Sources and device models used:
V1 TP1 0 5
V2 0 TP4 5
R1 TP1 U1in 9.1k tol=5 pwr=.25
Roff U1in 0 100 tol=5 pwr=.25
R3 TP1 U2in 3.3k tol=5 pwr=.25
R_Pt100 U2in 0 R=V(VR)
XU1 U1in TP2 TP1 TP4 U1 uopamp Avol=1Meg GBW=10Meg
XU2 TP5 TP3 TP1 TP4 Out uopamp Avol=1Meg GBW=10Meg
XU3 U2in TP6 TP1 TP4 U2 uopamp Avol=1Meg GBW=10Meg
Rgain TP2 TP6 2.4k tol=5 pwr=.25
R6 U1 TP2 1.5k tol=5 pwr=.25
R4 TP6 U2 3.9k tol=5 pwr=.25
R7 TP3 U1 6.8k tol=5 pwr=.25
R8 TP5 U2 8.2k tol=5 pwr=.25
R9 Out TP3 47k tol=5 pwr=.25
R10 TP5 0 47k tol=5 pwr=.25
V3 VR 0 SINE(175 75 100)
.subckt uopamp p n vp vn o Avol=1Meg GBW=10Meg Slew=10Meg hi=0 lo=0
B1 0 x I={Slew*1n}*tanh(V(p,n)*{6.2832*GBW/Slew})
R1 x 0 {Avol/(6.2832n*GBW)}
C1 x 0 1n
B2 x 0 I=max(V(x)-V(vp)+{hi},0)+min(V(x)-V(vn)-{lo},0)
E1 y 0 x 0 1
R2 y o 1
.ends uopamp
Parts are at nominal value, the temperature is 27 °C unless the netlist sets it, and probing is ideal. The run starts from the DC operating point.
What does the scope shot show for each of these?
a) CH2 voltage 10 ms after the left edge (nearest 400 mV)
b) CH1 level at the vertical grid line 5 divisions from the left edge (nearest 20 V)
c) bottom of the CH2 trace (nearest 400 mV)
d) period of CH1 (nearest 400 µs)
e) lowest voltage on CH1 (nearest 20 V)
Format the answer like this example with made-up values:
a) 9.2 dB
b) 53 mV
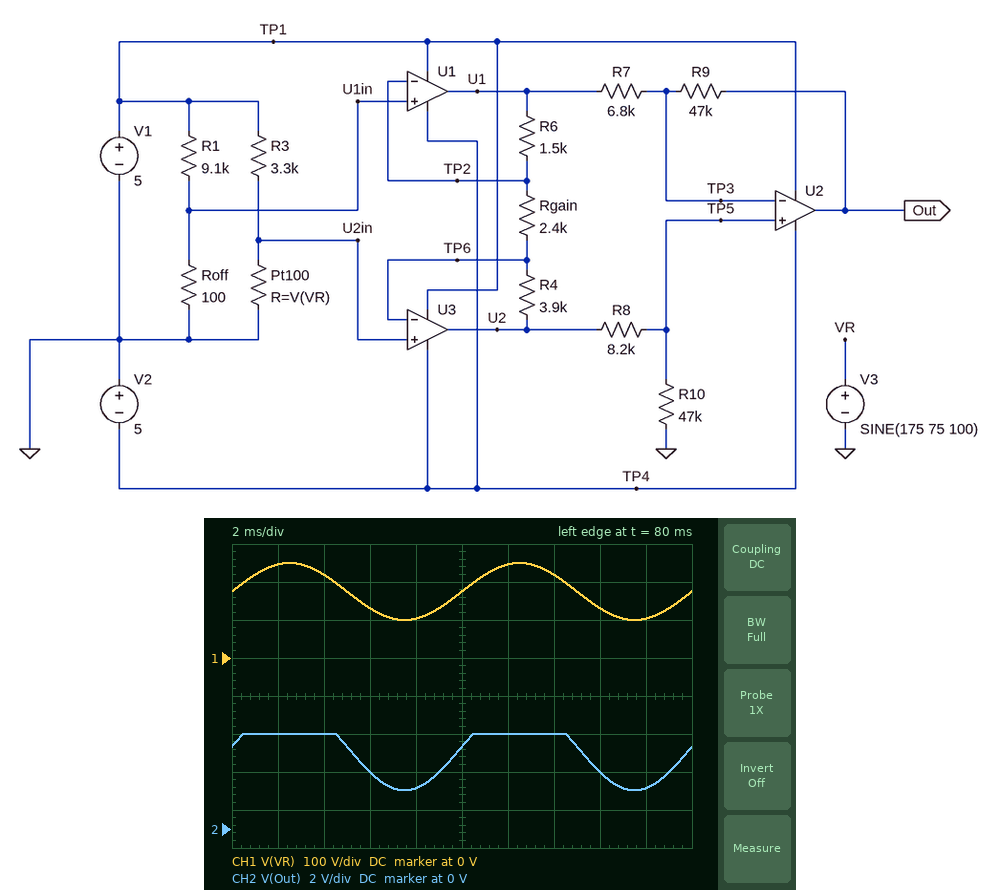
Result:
a) 4.4 V
b) 180 V
c) 2.0 V
d) 10.0 ms
e) 100 V
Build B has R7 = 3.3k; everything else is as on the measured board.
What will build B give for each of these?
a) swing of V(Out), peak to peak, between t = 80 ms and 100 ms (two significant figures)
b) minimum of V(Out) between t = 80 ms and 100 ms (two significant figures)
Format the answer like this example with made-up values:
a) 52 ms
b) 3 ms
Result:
a) 1.1 V
b) 3.9 V
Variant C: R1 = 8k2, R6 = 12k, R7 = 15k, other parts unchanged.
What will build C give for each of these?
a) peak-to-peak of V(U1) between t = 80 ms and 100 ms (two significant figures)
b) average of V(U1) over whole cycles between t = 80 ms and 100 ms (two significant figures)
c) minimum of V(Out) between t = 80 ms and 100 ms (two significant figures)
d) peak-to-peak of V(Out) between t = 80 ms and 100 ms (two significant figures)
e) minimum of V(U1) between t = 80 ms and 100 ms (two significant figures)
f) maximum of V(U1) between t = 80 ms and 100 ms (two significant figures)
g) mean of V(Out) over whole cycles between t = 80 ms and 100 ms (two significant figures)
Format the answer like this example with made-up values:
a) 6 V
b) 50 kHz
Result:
a) 1.0 V
b) -890 mV
c) 2.2 V
d) 2.8 V
e) -1.4 V
f) -370 mV
g) 4.1 V
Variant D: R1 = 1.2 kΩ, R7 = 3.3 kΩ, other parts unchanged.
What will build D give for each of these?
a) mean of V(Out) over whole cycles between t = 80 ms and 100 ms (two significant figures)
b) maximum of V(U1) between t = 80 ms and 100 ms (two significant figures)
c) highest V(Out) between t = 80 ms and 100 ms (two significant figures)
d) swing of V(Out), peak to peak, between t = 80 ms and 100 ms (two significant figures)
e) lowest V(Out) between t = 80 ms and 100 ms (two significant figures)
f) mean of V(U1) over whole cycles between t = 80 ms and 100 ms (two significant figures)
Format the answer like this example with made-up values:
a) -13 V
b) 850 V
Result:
a) -4.2 V
b) 530 mV
c) -1.9 V
d) 3.1 V
e) -5.0 V
f) 470 mV
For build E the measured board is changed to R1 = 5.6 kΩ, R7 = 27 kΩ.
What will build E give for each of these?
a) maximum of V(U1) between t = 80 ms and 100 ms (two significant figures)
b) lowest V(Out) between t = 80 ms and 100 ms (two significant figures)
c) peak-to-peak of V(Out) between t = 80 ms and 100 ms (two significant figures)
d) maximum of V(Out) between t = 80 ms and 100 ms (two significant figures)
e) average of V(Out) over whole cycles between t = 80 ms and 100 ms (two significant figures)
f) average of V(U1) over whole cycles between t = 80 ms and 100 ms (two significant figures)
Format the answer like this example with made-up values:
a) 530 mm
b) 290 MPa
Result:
a) 51 mV
b) 480 mV
c) 1.5 V
d) 2.0 V
e) 1.2 V
f) -14 mV
